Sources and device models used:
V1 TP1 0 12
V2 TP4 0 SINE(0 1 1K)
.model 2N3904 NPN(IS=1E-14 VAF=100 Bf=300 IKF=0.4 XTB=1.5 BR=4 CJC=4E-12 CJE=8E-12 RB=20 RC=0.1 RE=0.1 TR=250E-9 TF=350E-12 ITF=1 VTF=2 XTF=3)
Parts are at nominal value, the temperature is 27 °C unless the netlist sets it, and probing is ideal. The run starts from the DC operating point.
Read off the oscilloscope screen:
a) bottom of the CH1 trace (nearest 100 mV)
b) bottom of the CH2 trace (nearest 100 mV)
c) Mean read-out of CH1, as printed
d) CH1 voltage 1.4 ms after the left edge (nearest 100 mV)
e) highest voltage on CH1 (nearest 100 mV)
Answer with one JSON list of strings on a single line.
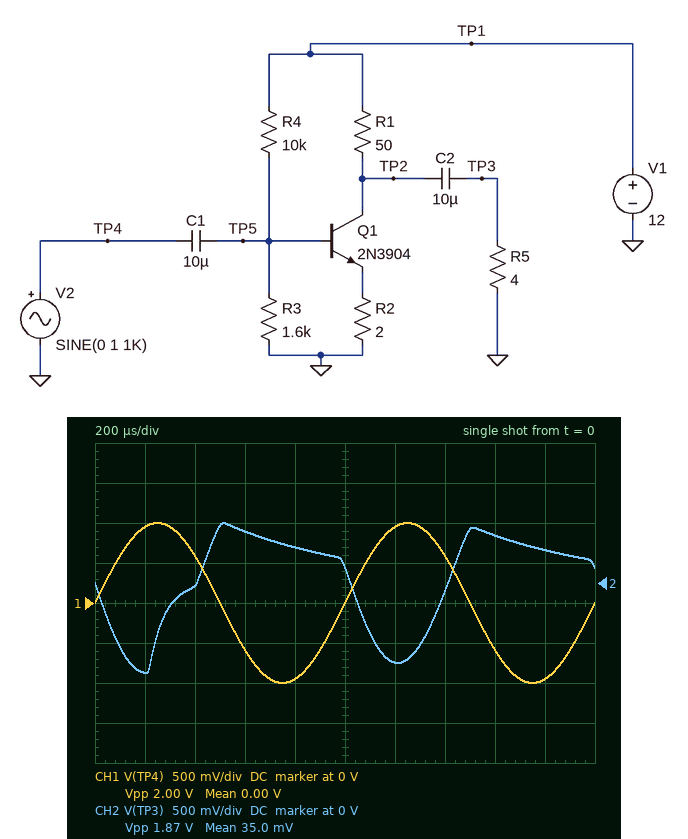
["-1.0 V", "-1.1 V", "0.00 V", "600 mV", "1.0 V"]
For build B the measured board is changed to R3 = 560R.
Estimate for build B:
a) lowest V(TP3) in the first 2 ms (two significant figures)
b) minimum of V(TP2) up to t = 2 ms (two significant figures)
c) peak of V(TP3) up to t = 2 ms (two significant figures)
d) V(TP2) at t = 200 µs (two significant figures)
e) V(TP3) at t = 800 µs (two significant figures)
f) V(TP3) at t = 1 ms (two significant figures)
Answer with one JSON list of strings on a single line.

["-1.0 V", "4.8 V", "480 mV", "8.1 V", "240 mV", "170 mV"]
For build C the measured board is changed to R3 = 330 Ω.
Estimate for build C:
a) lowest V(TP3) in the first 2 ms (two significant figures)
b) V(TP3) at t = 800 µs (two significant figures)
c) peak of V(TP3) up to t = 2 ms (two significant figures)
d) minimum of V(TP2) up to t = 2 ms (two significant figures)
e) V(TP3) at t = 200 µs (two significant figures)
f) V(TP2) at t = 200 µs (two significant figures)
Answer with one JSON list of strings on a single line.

["-720 mV", "140 mV", "300 mV", "7.5 V", "-710 mV", "9.7 V"]
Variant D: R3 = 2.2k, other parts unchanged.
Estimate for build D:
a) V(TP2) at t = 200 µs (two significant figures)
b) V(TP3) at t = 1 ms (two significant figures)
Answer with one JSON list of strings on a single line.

["960 mV", "220 mV"]
